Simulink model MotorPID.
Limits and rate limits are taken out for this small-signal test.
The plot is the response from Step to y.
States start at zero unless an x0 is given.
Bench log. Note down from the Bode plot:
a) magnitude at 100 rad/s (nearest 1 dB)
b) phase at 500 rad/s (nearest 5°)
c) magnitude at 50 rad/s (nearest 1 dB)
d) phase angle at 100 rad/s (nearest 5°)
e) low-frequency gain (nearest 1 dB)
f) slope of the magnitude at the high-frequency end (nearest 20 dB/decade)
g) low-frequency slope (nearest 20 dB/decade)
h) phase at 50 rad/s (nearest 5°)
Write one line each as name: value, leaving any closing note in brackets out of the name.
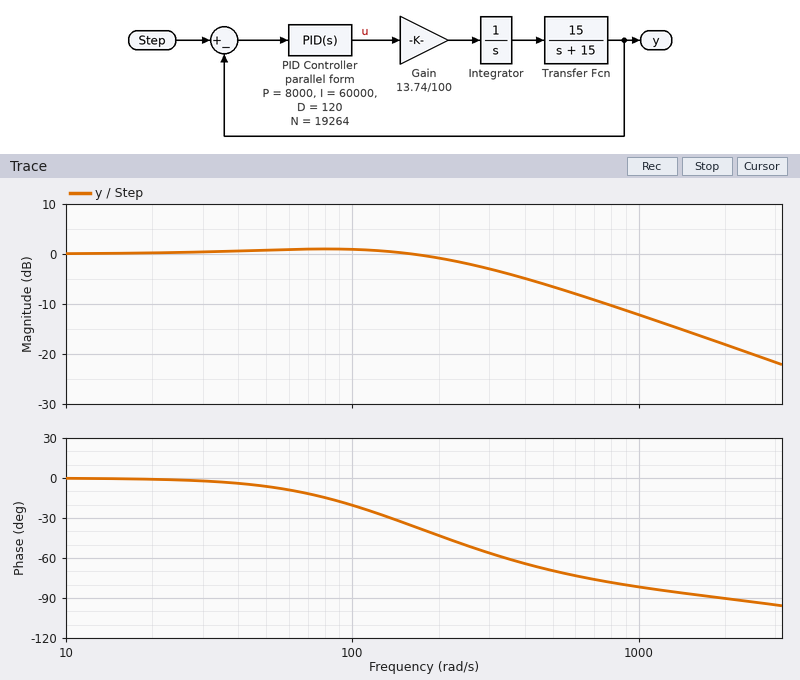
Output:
magnitude at 100 rad/s: 1 dB
phase at 500 rad/s: -70°
magnitude at 50 rad/s: 1 dB
phase angle at 100 rad/s: -20°
low-frequency gain: 0 dB
slope of the magnitude at the high-frequency end: -20 dB/decade
low-frequency slope: 0 dB/decade
phase at 50 rad/s: -5°
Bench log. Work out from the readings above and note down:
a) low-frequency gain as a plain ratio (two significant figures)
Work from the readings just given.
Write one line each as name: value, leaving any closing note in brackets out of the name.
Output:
low-frequency gain as a plain ratio: 1.0
